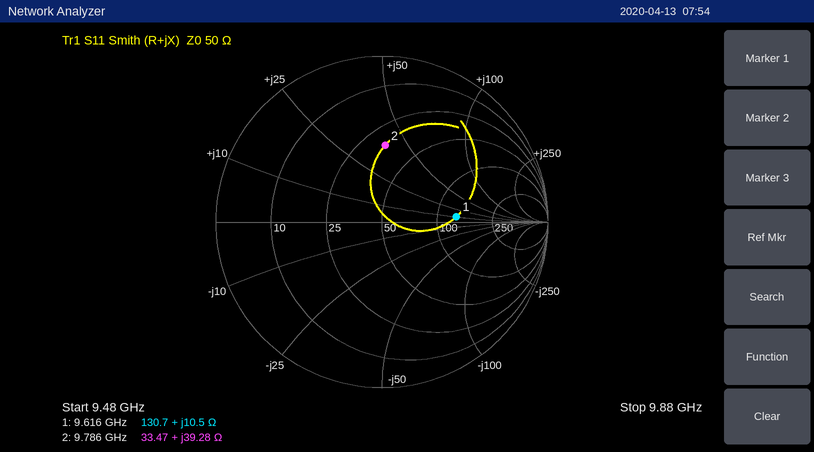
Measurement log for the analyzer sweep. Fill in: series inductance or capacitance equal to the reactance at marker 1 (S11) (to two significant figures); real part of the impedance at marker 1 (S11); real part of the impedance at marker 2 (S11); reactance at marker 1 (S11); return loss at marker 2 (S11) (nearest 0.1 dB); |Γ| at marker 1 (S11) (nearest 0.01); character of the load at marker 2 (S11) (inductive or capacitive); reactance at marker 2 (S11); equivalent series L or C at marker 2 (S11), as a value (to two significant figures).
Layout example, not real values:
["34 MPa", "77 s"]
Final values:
["170 pH", "130.7 Ω", "33.47 Ω", "+10.5 Ω", "6.7 dB", "0.45", "inductive", "+39.28 Ω", "640 pH"]
